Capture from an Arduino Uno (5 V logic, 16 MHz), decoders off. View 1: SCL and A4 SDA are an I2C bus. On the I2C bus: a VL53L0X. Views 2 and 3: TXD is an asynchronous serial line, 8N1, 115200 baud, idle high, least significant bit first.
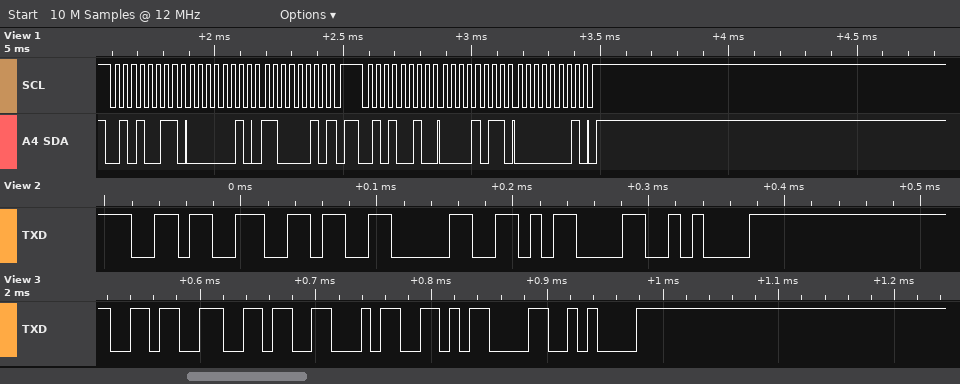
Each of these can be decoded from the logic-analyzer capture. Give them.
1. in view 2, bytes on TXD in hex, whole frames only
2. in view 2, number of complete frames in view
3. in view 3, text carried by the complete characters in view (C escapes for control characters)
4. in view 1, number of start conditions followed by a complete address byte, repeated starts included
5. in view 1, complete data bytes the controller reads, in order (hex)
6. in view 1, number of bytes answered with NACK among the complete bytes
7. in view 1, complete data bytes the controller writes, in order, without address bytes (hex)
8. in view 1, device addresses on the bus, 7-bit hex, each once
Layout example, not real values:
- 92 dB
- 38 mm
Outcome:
- 36 36 30 0D 0A
- 5
- "664\r\n"
- 2
- 02 C2
- 1
- 0B 01
- 0x29
